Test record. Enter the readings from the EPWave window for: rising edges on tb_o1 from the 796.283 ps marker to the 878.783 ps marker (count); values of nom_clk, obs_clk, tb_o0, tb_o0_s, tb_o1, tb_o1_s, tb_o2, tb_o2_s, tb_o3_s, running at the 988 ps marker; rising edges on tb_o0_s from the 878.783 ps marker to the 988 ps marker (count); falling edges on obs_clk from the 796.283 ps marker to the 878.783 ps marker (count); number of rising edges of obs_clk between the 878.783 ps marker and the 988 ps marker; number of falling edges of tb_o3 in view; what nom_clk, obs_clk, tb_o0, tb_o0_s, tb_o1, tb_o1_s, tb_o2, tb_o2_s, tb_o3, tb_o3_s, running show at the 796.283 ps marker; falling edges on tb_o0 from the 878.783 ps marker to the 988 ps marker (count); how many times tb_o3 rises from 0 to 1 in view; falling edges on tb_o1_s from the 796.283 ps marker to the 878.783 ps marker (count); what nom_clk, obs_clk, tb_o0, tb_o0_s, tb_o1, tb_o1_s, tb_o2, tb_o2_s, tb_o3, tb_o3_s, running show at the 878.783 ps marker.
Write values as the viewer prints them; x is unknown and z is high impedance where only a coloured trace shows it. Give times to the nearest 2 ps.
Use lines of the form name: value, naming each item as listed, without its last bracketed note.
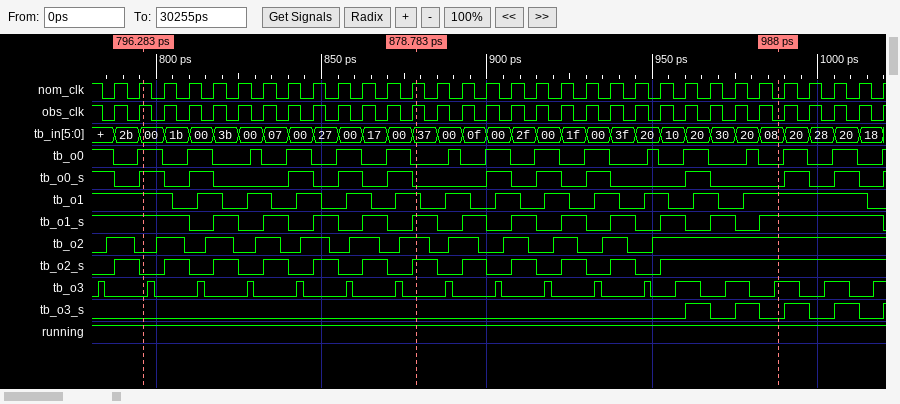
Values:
rising edges on tb_o1 from the 796.283 ps marker to the 878.783 ps marker: 5
values of nom_clk, obs_clk, tb_o0, tb_o0_s, tb_o1, tb_o1_s, tb_o2, tb_o2_s, tb_o3_s, running at the 988 ps marker: nom_clk=0, obs_clk=0, tb_o0=0, tb_o0_s=0, tb_o1=1, tb_o1_s=1, tb_o2=1, tb_o2_s=1, tb_o3_s=0, running=1
rising edges on tb_o0_s from the 878.783 ps marker to the 988 ps marker: 4
falling edges on obs_clk from the 796.283 ps marker to the 878.783 ps marker: 11
number of rising edges of obs_clk between the 878.783 ps marker and the 988 ps marker: 14
number of falling edges of tb_o3 in view: 16
what nom_clk, obs_clk, tb_o0, tb_o0_s, tb_o1, tb_o1_s, tb_o2, tb_o2_s, tb_o3, tb_o3_s, running show at the 796.283 ps marker: nom_clk=1, obs_clk=1, tb_o0=1, tb_o0_s=1, tb_o1=1, tb_o1_s=1, tb_o2=0, tb_o2_s=0, tb_o3=0, tb_o3_s=0, running=1
falling edges on tb_o0 from the 878.783 ps marker to the 988 ps marker: 7
how many times tb_o3 rises from 0 to 1 in view: 17
falling edges on tb_o1_s from the 796.283 ps marker to the 878.783 ps marker: 5
what nom_clk, obs_clk, tb_o0, tb_o0_s, tb_o1, tb_o1_s, tb_o2, tb_o2_s, tb_o3, tb_o3_s, running show at the 878.783 ps marker: nom_clk=1, obs_clk=1, tb_o0=0, tb_o0_s=0, tb_o1=1, tb_o1_s=1, tb_o2=1, tb_o2_s=1, tb_o3=0, tb_o3_s=0, running=1
